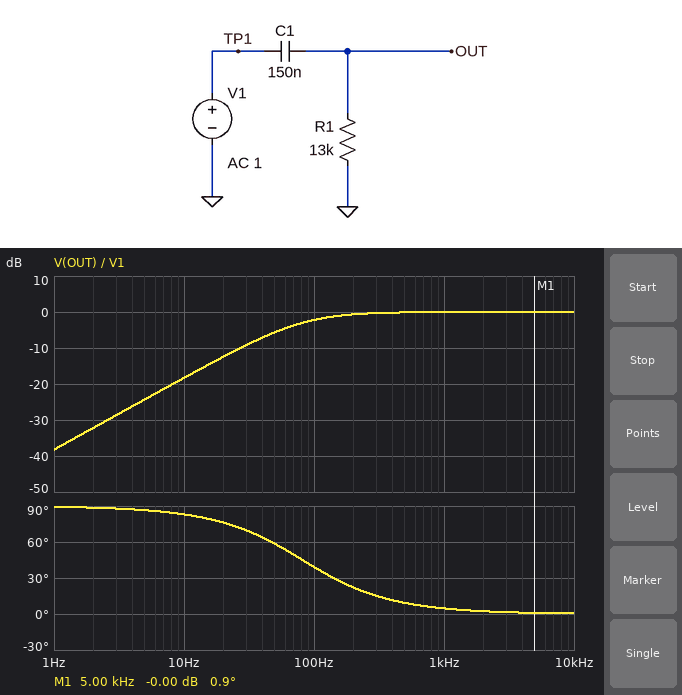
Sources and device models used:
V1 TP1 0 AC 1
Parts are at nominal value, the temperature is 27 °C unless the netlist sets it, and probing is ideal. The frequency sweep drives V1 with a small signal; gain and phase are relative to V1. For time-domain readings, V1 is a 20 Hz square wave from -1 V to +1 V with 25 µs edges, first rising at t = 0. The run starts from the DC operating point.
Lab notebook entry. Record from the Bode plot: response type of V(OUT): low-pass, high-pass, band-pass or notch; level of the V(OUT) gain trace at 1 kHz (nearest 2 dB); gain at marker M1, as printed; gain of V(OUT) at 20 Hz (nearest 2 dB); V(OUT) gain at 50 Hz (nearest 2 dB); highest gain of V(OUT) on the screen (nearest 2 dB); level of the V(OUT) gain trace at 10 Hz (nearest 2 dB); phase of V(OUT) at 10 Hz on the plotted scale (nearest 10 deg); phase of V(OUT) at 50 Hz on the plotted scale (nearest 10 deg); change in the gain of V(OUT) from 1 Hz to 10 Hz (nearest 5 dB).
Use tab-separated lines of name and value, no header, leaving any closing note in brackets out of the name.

response type of V(OUT): low-pass, high-pass, band-pass or notch	high-pass
level of the V(OUT) gain trace at 1 kHz	0 dB
gain at marker M1, as printed	-0.00 dB
gain of V(OUT) at 20 Hz	-12 dB
V(OUT) gain at 50 Hz	-6 dB
highest gain of V(OUT) on the screen	0 dB
level of the V(OUT) gain trace at 10 Hz	-18 dB
phase of V(OUT) at 10 Hz on the plotted scale	80 deg
phase of V(OUT) at 50 Hz on the plotted scale	60 deg
change in the gain of V(OUT) from 1 Hz to 10 Hz	20 dB
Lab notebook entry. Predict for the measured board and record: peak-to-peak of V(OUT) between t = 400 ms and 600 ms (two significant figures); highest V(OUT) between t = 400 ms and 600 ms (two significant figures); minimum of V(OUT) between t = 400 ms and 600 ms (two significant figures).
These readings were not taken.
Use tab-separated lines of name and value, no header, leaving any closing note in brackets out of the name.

peak-to-peak of V(OUT) between t = 400 ms and 600 ms	4.0 V
highest V(OUT) between t = 400 ms and 600 ms	2.0 V
minimum of V(OUT) between t = 400 ms and 600 ms	-2.0 V
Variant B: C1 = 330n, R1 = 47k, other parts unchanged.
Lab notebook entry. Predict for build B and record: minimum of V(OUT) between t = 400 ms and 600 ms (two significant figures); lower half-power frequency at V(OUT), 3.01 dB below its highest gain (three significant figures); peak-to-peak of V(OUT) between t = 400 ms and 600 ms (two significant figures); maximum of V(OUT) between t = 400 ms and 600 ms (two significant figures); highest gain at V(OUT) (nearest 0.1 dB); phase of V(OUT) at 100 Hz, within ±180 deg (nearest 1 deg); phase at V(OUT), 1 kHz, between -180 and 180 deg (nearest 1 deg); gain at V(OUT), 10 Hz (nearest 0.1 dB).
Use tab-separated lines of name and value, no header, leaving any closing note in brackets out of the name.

minimum of V(OUT) between t = 400 ms and 600 ms	-1.7 V
lower half-power frequency at V(OUT), 3.01 dB below its highest gain	10.3 Hz
peak-to-peak of V(OUT) between t = 400 ms and 600 ms	3.3 V
maximum of V(OUT) between t = 400 ms and 600 ms	1.7 V
highest gain at V(OUT)	0 dB
phase of V(OUT) at 100 Hz, within ±180 deg	6 deg
phase at V(OUT), 1 kHz, between -180 and 180 deg	1 deg
gain at V(OUT), 10 Hz	-3.1 dB
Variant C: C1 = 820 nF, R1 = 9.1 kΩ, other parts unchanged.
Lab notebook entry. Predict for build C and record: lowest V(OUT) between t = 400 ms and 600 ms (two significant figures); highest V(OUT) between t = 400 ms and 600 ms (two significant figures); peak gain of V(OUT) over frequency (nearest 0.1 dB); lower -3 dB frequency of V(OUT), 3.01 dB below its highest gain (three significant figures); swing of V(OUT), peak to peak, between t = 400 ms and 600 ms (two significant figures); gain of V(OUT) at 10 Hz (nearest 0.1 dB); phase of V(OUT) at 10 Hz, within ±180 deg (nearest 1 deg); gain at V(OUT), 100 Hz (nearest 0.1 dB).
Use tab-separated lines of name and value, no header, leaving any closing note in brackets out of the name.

lowest V(OUT) between t = 400 ms and 600 ms	-1.9 V
highest V(OUT) between t = 400 ms and 600 ms	1.9 V
peak gain of V(OUT) over frequency	0 dB
lower -3 dB frequency of V(OUT), 3.01 dB below its highest gain	21.3 Hz
swing of V(OUT), peak to peak, between t = 400 ms and 600 ms	3.9 V
gain of V(OUT) at 10 Hz	-7.4 dB
phase of V(OUT) at 10 Hz, within ±180 deg	65 deg
gain at V(OUT), 100 Hz	-0.2 dB
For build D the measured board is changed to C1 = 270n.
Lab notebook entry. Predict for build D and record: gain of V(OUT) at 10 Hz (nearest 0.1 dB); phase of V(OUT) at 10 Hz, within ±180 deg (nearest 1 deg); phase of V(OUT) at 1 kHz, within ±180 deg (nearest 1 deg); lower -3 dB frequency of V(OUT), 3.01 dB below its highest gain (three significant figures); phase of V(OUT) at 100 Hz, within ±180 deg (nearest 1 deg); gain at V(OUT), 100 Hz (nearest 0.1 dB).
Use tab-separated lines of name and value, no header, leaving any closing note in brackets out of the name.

gain of V(OUT) at 10 Hz	-13.3 dB
phase of V(OUT) at 10 Hz, within ±180 deg	78 deg
phase of V(OUT) at 1 kHz, within ±180 deg	3 deg
lower -3 dB frequency of V(OUT), 3.01 dB below its highest gain	45.3 Hz
phase of V(OUT) at 100 Hz, within ±180 deg	24 deg
gain at V(OUT), 100 Hz	-0.8 dB
